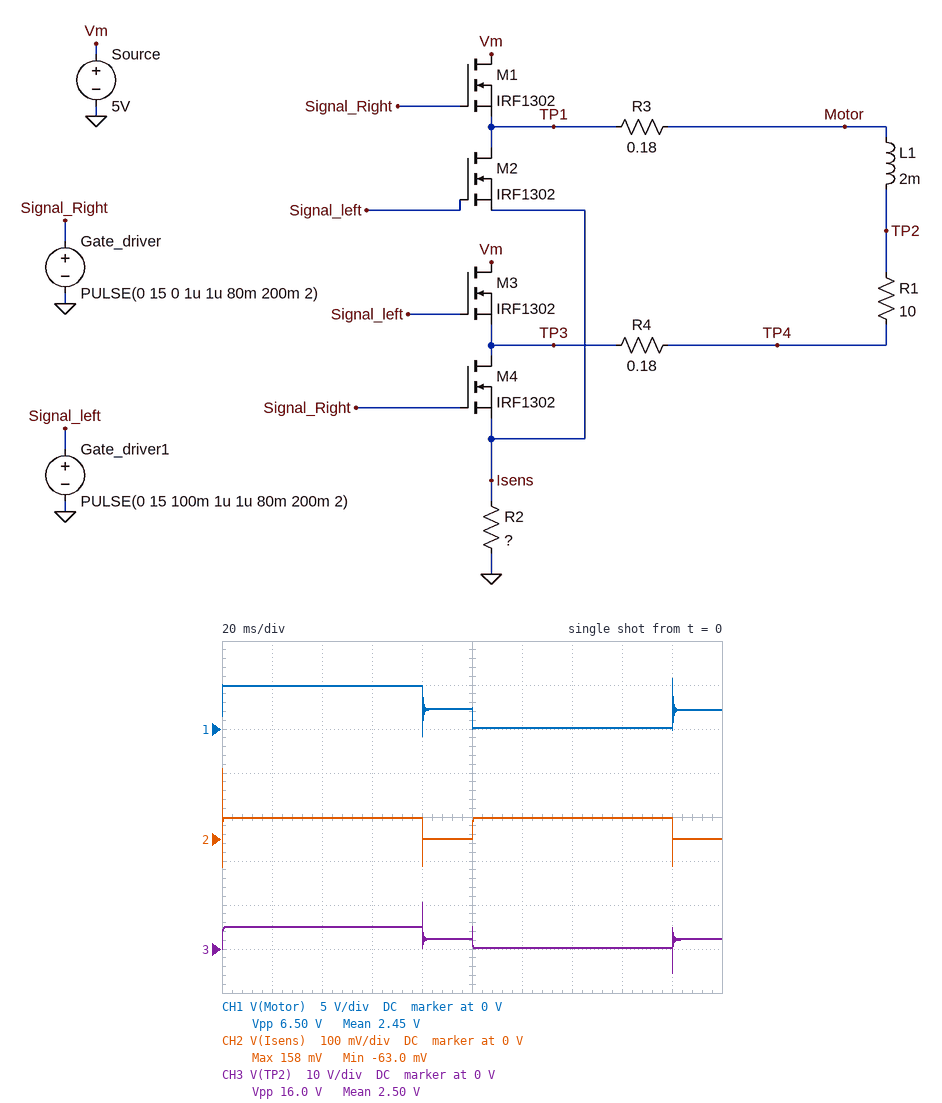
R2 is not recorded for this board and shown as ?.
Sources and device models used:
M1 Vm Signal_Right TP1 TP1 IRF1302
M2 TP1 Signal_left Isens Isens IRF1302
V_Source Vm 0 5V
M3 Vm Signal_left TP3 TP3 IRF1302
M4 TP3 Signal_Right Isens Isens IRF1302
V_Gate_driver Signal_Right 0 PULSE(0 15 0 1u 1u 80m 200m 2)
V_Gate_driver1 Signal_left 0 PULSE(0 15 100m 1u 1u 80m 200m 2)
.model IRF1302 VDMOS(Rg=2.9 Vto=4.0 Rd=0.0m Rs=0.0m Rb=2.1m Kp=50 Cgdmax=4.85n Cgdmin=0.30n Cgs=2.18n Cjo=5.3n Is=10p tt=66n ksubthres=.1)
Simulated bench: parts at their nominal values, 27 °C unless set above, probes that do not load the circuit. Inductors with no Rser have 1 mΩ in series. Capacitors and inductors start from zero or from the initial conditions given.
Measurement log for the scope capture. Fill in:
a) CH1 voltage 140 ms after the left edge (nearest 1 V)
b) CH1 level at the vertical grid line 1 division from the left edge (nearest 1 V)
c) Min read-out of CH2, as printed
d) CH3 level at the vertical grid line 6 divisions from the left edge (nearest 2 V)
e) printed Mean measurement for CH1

0 V
5 V
-63.0 mV
0 V
2.45 V
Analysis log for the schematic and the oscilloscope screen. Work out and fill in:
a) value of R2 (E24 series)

0.1 Ω
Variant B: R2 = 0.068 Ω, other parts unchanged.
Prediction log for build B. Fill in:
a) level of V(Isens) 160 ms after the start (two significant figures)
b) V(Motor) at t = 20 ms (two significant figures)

33 mV
4.9 V
